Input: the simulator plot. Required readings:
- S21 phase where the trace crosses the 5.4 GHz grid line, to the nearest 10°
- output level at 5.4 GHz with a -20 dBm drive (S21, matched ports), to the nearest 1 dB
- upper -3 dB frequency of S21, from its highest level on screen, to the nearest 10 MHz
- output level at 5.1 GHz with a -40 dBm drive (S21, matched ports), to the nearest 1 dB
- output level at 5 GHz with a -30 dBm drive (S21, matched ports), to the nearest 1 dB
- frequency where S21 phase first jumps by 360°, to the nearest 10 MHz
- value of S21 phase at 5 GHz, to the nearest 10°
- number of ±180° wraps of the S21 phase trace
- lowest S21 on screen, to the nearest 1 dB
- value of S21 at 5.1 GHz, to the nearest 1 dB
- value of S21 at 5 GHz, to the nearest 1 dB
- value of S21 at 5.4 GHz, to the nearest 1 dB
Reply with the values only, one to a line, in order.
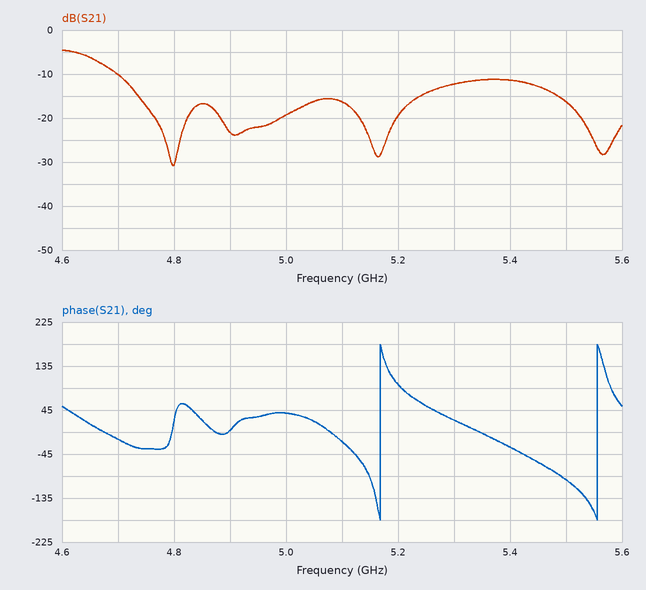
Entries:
-30°
-31 dBm
4.67 GHz
-56 dBm
-49 dBm
5.17 GHz
40°
2
-31 dB
-16 dB
-19 dB
-11 dB
